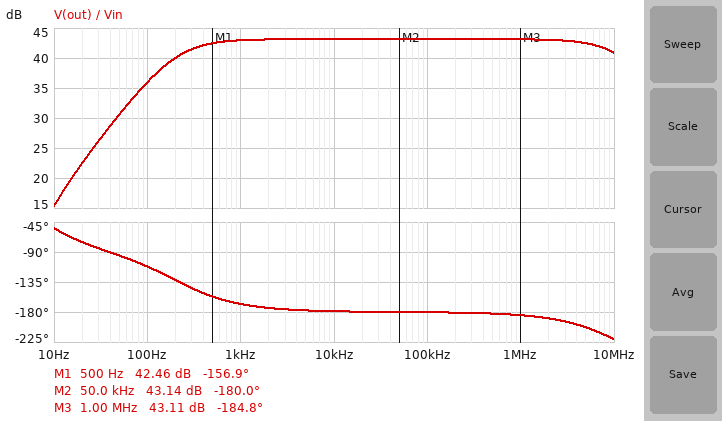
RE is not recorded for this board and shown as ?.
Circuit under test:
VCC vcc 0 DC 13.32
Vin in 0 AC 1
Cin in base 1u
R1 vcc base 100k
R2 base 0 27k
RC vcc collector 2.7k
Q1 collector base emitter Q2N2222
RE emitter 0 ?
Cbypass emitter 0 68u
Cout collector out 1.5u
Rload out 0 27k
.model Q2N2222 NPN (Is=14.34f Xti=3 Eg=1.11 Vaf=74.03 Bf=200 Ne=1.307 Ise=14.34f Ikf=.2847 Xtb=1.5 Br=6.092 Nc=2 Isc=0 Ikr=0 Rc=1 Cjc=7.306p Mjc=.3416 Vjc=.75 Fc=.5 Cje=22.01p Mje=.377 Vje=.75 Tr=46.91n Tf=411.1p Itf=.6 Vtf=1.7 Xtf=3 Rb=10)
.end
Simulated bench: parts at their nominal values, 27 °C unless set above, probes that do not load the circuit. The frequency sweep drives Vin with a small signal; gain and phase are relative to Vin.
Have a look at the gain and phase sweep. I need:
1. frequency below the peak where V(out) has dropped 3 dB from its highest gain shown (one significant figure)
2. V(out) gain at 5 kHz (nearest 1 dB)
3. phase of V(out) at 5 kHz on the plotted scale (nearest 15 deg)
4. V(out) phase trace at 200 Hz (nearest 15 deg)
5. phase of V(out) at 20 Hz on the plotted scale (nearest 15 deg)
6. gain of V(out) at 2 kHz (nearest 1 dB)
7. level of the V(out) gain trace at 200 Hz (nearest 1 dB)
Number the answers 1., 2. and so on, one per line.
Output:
1. 200 Hz
2. 43 dB
3. -180 deg
4. -135 deg
5. -75 deg
6. 43 dB
7. 40 dB
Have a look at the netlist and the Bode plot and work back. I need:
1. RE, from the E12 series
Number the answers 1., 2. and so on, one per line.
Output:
1. 1.2 kΩ
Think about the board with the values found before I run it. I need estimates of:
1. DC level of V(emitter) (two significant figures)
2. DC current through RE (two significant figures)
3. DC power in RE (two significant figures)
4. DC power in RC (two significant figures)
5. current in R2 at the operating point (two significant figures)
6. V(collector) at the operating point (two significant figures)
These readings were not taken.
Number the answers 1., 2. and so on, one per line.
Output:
1. 1.9 V
2. 1.6 mA
3. 3.1 mW
4. 6.9 mW
5. 96 µA
6. 9.0 V
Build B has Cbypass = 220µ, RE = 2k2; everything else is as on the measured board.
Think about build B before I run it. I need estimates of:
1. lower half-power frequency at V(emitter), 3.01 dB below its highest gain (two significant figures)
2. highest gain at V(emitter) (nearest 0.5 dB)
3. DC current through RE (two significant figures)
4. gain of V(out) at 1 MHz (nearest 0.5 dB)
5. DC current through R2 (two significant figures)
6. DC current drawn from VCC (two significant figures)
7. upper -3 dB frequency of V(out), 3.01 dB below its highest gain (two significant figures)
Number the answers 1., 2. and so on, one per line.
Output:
1. 2.8 Hz
2. -9.0 dB
3. 930 µA
4. 38.5 dB
5. 100 µA
6. 1.0 mA
7. 15 MHz
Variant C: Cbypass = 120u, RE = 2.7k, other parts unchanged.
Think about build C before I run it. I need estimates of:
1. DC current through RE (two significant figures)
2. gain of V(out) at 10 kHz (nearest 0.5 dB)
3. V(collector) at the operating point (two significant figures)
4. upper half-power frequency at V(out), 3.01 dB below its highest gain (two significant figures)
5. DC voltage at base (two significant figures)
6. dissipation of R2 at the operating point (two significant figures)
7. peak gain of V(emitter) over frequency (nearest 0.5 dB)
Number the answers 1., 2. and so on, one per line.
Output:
1. 770 µA
2. 37.0 dB
3. 11 V
4. 16 MHz
5. 2.7 V
6. 270 µW
7. -6.0 dB
